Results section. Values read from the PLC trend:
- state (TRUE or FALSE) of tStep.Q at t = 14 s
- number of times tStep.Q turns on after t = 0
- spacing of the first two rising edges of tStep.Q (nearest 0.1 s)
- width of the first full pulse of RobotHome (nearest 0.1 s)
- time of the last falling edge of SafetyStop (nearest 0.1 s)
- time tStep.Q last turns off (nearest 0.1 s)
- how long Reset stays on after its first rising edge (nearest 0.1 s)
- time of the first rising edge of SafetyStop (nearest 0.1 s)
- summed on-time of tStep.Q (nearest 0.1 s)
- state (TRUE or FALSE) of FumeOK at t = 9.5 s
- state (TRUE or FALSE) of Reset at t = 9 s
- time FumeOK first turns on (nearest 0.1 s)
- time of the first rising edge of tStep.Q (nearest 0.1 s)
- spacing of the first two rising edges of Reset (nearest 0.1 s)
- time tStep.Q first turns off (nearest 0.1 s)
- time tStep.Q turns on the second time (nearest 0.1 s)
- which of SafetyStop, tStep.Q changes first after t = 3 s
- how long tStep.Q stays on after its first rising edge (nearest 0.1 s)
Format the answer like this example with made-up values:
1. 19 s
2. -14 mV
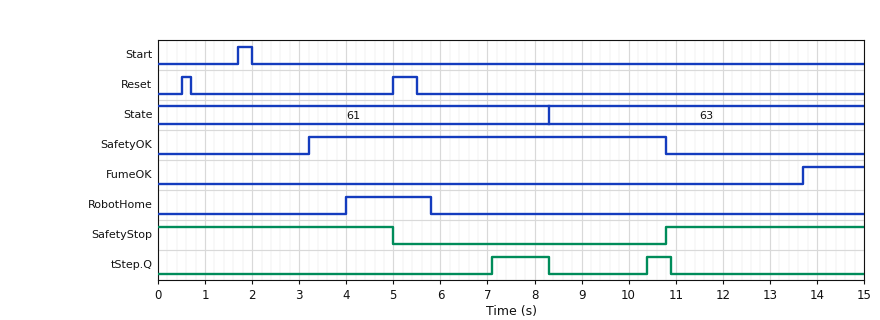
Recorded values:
1. FALSE
2. 2
3. 3.3 s
4. 1.8 s
5. 5.0 s
6. 10.9 s
7. 0.2 s
8. 10.8 s
9. 1.7 s
10. FALSE
11. FALSE
12. 13.7 s
13. 7.1 s
14. 4.5 s
15. 8.3 s
16. 10.4 s
17. SafetyStop
18. 1.2 s
